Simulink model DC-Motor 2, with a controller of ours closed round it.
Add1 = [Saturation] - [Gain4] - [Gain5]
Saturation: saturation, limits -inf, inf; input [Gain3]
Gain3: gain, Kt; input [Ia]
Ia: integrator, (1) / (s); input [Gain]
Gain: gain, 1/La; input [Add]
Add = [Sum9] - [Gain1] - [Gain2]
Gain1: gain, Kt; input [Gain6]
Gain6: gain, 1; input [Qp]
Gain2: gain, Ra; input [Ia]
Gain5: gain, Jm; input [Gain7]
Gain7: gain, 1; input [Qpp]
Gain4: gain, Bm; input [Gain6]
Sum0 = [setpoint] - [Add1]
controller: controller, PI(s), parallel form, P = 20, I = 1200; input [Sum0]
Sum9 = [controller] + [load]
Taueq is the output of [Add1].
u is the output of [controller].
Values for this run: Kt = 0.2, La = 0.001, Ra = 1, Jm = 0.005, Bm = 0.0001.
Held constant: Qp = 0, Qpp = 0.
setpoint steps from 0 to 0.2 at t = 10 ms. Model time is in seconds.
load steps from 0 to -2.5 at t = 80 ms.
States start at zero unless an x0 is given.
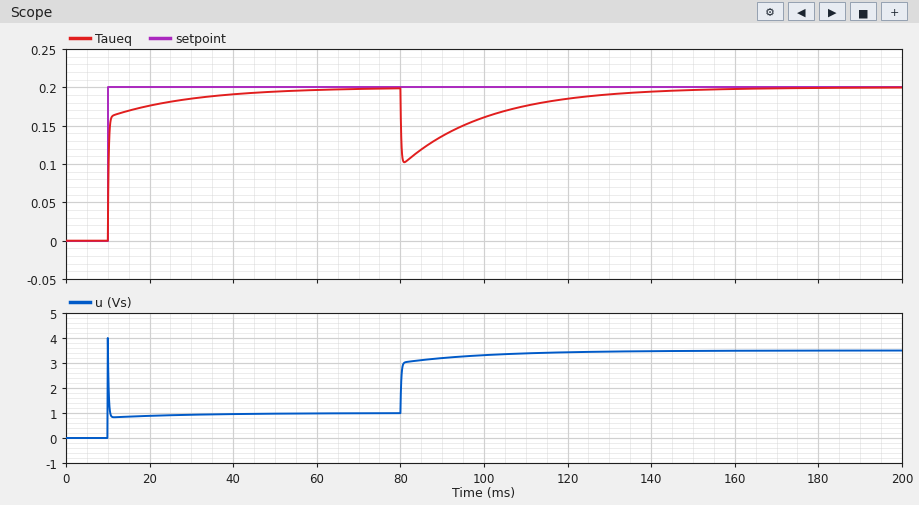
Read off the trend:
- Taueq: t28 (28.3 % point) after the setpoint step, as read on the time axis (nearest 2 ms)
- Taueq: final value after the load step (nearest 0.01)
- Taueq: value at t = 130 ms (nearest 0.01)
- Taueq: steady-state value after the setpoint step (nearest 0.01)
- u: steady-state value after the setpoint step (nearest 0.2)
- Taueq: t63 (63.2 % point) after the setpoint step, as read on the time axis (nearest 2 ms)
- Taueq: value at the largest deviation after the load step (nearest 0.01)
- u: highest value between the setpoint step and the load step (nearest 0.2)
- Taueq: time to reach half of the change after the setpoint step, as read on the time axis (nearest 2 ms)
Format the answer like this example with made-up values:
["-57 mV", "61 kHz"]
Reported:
["10 ms", "0.20", "0.19", "0.20", "1.0", "10 ms", "0.10", "4.0", "10 ms"]
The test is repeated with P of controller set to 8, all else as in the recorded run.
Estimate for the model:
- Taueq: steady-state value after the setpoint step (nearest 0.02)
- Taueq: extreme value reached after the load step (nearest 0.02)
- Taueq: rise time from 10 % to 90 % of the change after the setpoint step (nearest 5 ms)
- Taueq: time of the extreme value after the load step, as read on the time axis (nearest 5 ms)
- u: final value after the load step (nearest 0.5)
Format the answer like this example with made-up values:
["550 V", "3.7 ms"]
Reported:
["0.20", "0.02", "15 ms", "80 ms", "3.5"]
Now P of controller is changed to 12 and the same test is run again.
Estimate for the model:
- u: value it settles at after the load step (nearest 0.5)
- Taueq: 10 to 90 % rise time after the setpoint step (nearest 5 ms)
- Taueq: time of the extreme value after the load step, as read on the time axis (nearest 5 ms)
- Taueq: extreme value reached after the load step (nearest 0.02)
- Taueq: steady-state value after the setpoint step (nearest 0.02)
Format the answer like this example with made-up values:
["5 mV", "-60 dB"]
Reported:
["3.5", "15 ms", "80 ms", "0.06", "0.20"]
